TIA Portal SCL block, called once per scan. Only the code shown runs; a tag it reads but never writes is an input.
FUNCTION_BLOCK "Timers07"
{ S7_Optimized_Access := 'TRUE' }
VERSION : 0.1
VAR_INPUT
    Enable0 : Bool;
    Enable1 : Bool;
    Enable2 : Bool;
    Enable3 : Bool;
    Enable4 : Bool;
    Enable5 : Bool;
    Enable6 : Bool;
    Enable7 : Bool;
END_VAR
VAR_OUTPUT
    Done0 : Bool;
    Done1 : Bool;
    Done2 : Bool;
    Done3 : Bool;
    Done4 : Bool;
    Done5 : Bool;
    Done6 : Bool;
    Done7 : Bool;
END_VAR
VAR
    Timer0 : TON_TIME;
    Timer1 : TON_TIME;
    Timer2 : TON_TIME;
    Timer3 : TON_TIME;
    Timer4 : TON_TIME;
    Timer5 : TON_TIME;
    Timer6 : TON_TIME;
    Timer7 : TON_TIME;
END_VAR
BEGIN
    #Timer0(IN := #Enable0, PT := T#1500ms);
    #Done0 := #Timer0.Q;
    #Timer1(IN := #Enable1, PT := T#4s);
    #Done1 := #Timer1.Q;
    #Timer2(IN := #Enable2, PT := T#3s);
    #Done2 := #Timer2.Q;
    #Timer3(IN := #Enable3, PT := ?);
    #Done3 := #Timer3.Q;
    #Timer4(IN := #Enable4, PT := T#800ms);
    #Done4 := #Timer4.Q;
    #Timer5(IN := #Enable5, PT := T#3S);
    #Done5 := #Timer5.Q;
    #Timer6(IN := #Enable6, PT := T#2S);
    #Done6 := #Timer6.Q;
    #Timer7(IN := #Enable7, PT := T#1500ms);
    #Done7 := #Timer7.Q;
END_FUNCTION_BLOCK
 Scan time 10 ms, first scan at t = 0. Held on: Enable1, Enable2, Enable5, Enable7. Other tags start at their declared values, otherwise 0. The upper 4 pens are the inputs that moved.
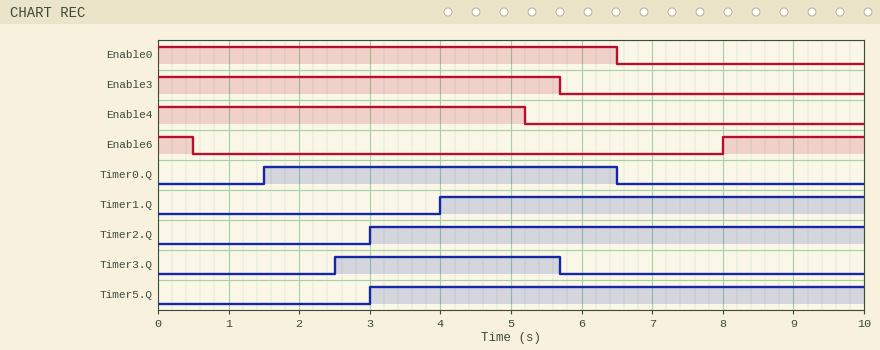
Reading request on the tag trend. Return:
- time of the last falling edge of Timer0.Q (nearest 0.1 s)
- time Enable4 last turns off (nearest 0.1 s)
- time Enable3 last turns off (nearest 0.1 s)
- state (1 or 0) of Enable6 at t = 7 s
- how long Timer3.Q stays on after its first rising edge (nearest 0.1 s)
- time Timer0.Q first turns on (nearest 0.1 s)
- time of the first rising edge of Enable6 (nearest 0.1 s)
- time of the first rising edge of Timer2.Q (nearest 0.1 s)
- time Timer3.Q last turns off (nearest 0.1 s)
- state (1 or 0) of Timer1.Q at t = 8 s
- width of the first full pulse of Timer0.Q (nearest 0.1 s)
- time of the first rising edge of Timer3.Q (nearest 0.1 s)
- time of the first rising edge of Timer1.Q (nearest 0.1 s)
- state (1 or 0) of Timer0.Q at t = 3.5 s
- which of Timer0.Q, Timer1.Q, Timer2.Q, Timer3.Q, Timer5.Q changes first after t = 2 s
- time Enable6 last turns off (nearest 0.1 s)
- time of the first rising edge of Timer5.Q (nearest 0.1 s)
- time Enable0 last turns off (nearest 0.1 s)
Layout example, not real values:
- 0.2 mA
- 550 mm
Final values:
- 6.5 s
- 5.2 s
- 5.7 s
- 0
- 3.2 s
- 1.5 s
- 8.0 s
- 3.0 s
- 5.7 s
- 1
- 5.0 s
- 2.5 s
- 4.0 s
- 1
- Timer3.Q
- 0.5 s
- 3.0 s
- 6.5 s
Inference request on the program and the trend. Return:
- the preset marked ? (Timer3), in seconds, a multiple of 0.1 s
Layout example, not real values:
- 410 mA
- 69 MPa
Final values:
- 2.5 s
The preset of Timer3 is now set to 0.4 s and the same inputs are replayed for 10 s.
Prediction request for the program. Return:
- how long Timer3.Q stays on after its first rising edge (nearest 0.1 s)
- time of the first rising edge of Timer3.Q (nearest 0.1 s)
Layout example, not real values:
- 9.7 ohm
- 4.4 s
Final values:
- 5.3 s
- 0.4 s
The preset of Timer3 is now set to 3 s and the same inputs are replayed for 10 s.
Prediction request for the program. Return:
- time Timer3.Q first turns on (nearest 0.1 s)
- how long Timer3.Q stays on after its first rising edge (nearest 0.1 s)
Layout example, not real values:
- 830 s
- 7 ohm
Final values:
- 3.0 s
- 2.7 s
